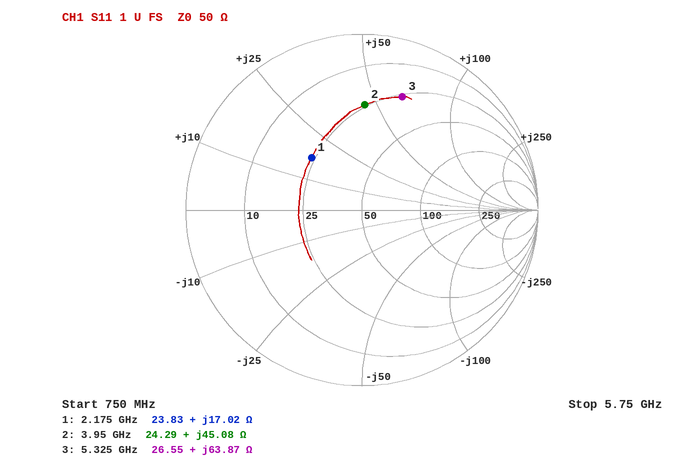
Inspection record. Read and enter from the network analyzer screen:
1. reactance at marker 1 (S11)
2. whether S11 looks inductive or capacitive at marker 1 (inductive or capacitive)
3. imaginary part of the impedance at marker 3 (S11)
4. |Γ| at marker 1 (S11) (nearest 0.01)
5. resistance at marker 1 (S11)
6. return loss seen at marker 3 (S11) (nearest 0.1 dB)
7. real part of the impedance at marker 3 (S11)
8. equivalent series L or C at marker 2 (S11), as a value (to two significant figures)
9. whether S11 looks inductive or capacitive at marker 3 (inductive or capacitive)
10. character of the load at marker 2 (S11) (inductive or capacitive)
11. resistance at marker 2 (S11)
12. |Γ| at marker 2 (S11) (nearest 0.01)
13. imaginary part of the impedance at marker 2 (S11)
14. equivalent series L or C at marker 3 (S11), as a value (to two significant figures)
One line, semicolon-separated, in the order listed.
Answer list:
+17.02 Ω; inductive; +63.87 Ω; 0.41; 23.83 Ω; 3.3 dB; 26.55 Ω; 1.8 nH; inductive; inductive; 24.29 Ω; 0.60; +45.08 Ω; 1.9 nH
